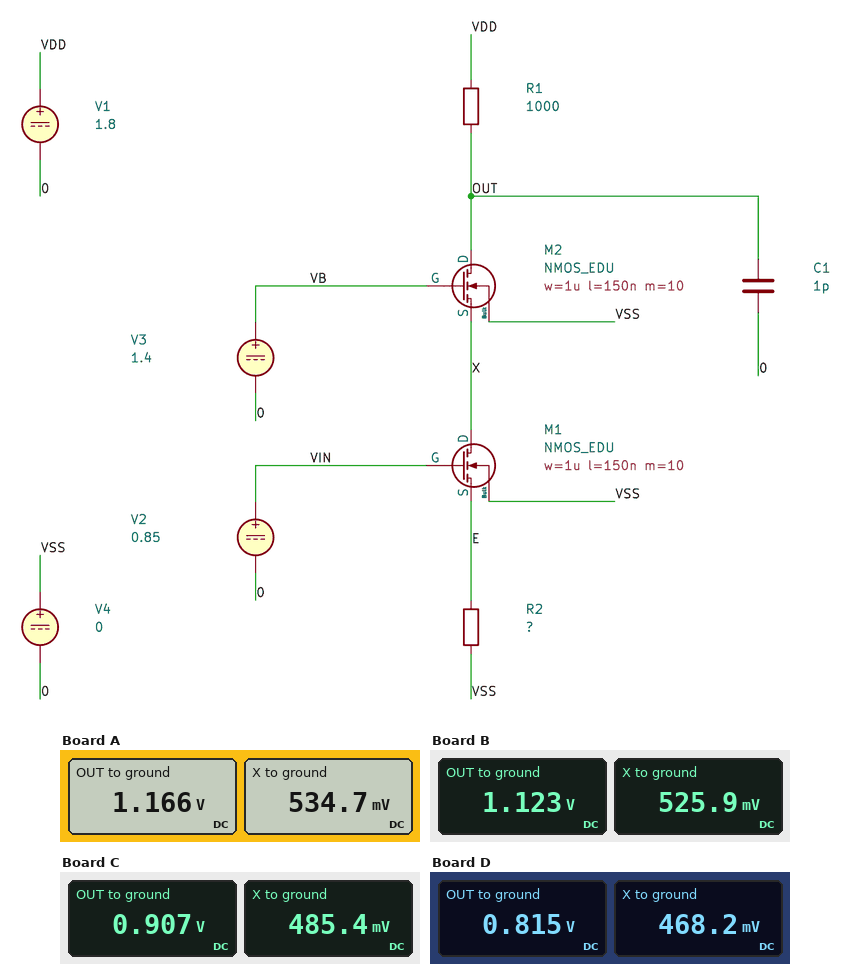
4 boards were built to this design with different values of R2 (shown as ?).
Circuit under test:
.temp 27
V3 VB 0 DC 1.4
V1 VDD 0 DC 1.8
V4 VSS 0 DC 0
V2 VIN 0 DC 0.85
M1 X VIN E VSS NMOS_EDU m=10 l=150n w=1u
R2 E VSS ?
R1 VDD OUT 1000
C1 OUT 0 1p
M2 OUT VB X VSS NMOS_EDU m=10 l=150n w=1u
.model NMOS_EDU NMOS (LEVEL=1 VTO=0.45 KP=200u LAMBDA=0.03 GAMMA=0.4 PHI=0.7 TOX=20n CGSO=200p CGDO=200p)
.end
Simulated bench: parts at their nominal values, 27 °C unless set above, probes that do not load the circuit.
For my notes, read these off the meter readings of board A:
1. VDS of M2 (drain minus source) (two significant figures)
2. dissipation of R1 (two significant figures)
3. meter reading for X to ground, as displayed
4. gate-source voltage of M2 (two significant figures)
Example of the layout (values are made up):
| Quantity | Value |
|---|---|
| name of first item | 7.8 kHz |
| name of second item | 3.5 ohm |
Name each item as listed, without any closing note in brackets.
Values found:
| Quantity | Value |
|---|---|
| VDS of M2 (drain minus source) | 630 mV |
| dissipation of R1 | 400 µW |
| meter reading for X to ground, as displayed | 534.7 mV |
| gate-source voltage of M2 | 870 mV |
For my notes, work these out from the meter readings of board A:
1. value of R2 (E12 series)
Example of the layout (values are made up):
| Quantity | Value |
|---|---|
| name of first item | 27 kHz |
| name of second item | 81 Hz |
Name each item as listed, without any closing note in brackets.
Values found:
| Quantity | Value |
|---|---|
| value of R2 | 120 Ω |
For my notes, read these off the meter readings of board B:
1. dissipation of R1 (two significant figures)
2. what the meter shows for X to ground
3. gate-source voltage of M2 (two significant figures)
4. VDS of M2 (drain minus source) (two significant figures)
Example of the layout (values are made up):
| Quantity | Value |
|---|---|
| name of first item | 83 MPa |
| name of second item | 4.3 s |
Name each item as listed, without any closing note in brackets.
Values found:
| Quantity | Value |
|---|---|
| dissipation of R1 | 460 µW |
| what the meter shows for X to ground | 525.9 mV |
| gate-source voltage of M2 | 870 mV |
| VDS of M2 (drain minus source) | 600 mV |
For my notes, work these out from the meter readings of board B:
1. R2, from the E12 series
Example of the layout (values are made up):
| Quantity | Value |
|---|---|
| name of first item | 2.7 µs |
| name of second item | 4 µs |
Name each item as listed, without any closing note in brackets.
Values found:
| Quantity | Value |
|---|---|
| R2, from the E12 series | 100 Ω |
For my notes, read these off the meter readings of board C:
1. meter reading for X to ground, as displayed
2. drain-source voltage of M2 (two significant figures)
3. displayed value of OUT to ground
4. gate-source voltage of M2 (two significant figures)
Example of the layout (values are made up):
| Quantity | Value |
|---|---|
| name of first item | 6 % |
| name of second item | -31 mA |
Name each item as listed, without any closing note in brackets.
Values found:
| Quantity | Value |
|---|---|
| meter reading for X to ground, as displayed | 485.4 mV |
| drain-source voltage of M2 | 420 mV |
| displayed value of OUT to ground | 0.907 V |
| gate-source voltage of M2 | 910 mV |
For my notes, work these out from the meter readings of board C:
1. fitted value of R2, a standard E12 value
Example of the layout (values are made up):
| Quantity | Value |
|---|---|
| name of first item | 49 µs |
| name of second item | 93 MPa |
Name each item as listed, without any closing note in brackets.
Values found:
| Quantity | Value |
|---|---|
| fitted value of R2, a standard E12 value | 33 Ω |
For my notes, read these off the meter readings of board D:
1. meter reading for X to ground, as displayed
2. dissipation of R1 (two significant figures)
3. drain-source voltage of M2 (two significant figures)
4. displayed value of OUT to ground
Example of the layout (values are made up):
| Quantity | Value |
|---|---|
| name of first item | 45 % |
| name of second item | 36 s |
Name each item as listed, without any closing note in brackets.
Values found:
| Quantity | Value |
|---|---|
| meter reading for X to ground, as displayed | 468.2 mV |
| dissipation of R1 | 970 µW |
| drain-source voltage of M2 | 350 mV |
| displayed value of OUT to ground | 0.815 V |
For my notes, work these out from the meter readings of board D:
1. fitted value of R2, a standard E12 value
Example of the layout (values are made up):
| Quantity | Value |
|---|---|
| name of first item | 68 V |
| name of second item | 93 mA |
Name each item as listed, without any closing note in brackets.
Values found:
| Quantity | Value |
|---|---|
| fitted value of R2, a standard E12 value | 15 Ω |
